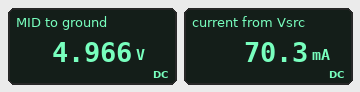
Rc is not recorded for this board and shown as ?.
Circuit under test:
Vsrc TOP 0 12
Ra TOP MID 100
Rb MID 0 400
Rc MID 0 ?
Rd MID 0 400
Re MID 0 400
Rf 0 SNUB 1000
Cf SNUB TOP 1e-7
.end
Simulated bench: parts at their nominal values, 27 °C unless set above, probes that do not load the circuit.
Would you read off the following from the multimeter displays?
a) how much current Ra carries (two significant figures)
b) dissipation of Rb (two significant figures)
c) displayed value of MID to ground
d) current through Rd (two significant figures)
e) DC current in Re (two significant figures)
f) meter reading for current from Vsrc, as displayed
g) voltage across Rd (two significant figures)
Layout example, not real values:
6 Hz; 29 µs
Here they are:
70 mA; 62 mW; 4.966 V; 12 mA; 12 mA; 70.3 mA; 5.0 V
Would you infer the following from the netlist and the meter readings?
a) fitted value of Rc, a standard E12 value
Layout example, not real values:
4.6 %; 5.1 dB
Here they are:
150 Ω
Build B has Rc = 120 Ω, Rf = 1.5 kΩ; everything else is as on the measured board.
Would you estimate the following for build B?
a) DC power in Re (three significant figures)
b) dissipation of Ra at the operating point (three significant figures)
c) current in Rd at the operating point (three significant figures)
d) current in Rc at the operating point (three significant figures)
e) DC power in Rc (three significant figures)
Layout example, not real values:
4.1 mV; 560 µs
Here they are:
53.9 mW; 541 mW; 11.6 mA; 38.7 mA; 180 mW
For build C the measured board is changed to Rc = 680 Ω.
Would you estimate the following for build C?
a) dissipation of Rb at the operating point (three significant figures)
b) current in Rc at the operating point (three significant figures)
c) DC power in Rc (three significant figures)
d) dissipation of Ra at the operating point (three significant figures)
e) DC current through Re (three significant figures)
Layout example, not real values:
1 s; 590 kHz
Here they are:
100 mW; 9.30 mA; 58.8 mW; 322 mW; 15.8 mA
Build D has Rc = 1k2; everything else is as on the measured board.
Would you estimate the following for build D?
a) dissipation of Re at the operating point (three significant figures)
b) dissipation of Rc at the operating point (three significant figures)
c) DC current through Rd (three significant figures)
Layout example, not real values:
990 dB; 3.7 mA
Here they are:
107 mW; 35.7 mW; 16.4 mA
